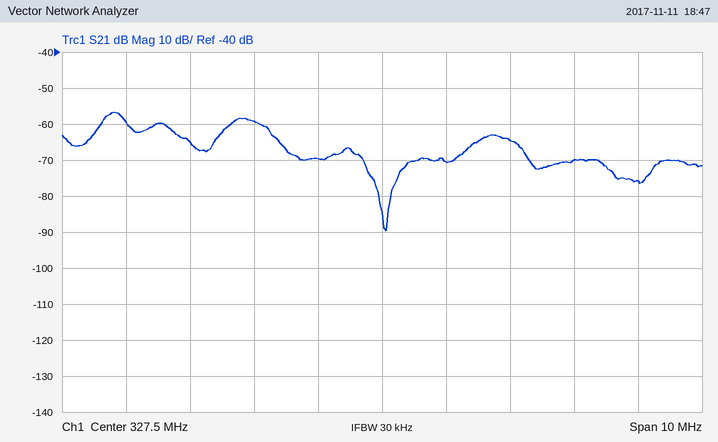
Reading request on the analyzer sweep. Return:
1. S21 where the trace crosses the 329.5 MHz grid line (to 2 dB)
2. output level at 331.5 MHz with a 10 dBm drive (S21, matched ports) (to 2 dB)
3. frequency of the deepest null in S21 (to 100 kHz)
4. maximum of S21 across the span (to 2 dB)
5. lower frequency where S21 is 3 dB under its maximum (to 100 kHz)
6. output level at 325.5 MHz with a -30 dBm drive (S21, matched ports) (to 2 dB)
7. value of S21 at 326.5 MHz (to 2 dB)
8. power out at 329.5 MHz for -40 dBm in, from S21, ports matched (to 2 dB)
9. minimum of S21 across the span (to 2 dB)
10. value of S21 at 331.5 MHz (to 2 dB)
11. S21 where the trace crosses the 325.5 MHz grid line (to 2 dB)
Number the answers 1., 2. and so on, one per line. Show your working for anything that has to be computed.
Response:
1. -64 dB
2. 10 dBm + (-76 dB) = -66 dBm
3. 327.6 MHz
4. -56 dB
5. 323.1 MHz
6. -30 dBm + (-60 dB) = -90 dBm
7. -70 dB
8. -40 dBm + (-64 dB) = -104 dBm
9. -90 dB
10. -76 dB
11. -60 dB
